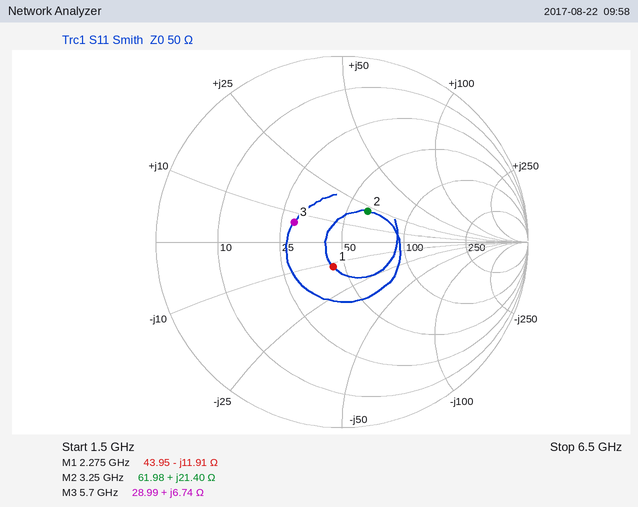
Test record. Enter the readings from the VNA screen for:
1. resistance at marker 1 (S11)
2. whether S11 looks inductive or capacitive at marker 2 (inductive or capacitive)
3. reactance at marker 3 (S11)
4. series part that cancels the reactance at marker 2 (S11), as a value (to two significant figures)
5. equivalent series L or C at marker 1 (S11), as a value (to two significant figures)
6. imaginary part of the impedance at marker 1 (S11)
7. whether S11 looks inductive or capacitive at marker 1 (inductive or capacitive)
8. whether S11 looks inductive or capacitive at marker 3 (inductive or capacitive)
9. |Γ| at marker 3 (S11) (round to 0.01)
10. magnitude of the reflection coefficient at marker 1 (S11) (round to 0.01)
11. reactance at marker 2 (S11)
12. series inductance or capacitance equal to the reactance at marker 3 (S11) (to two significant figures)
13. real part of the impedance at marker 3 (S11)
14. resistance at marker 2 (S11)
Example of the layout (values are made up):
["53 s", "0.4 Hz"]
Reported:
["43.95 Ω", "inductive", "+6.74 Ω", "2.3 pF", "5.9 pF", "-11.91 Ω", "capacitive", "inductive", "0.28", "0.14", "+21.40 Ω", "190 pH", "28.99 Ω", "61.98 Ω"]
